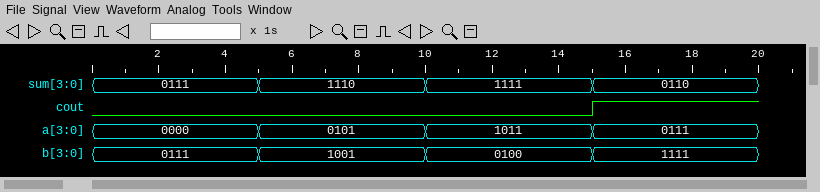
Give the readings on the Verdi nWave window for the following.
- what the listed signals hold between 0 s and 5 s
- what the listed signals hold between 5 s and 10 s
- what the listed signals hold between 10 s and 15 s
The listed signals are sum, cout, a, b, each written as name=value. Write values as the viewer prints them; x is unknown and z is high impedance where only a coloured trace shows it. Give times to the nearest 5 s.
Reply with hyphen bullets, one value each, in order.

- sum=0111, cout=0, a=0000, b=0111
- sum=1110, cout=0, a=0101, b=1001
- sum=1111, cout=0, a=1011, b=0100
